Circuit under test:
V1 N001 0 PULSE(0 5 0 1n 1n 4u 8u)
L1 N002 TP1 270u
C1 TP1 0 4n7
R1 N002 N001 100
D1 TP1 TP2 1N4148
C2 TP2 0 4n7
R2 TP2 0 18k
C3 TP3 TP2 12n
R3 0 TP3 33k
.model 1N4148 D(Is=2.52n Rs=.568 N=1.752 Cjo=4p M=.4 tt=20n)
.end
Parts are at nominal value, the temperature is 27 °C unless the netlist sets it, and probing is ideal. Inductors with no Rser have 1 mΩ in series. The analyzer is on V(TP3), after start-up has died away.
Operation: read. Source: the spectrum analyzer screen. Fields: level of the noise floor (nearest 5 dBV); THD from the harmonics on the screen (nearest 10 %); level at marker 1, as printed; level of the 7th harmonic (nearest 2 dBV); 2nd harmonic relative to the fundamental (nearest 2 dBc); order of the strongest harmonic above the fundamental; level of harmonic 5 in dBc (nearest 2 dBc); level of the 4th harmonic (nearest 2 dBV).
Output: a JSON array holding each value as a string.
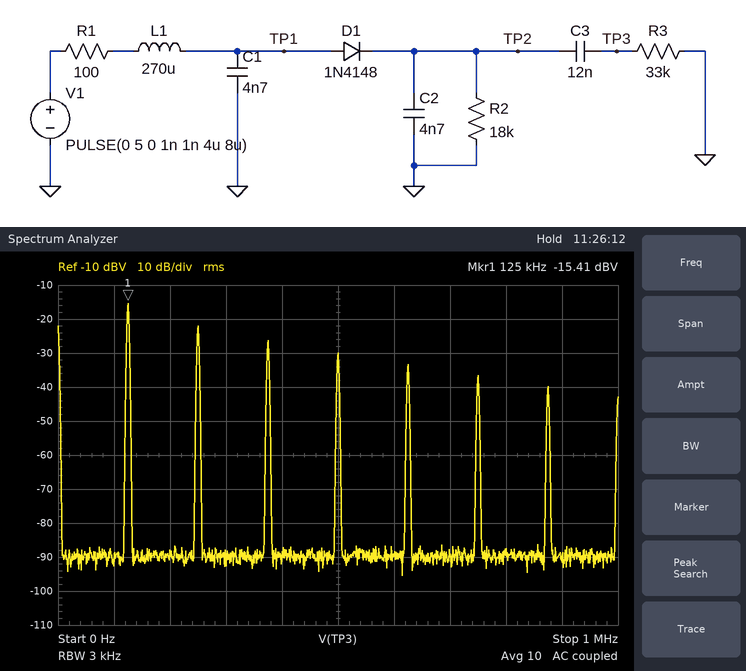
["-90 dBV", "60 %", "-15.41 dBV", "-40 dBV", "-6 dBc", "2", "-18 dBc", "-30 dBV"]
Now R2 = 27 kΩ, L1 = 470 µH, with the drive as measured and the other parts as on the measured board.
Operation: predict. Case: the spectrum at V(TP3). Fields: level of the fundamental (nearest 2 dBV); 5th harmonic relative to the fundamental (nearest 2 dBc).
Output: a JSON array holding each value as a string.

["-20 dBV", "-16 dBc"]
